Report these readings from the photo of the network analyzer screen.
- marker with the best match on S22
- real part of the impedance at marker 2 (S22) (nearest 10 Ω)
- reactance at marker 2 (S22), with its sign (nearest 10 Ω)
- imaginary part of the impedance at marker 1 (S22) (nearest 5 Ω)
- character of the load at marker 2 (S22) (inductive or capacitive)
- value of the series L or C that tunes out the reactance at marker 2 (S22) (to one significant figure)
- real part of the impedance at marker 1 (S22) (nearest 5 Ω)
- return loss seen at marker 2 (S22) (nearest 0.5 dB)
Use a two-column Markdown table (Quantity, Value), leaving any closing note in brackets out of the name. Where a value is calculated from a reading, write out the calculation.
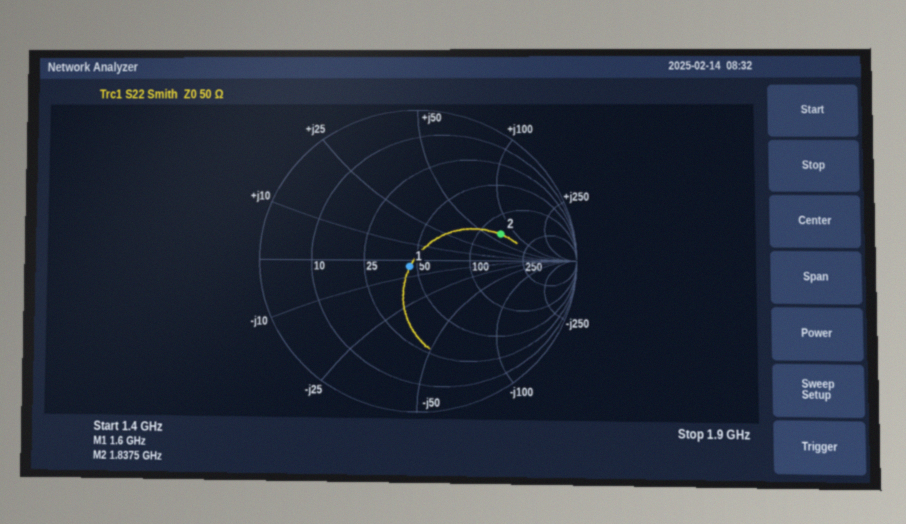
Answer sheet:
| Quantity | Value |
|---|---|
| marker with the best match on S22 | marker 1 |
| real part of the impedance at marker 2 (S22) | 140 Ω |
| reactance at marker 2 (S22), with its sign | +70 Ω |
| imaginary part of the impedance at marker 1 (S22) | -5 Ω |
| character of the load at marker 2 (S22) | inductive |
| value of the series L or C that tunes out the reactance at marker 2 (S22) | C = 1/(2π × 1.8375 GHz × 70 Ω) ≈ 1 pF |
| real part of the impedance at marker 1 (S22) | 45 Ω |
| return loss seen at marker 2 (S22) | 5.0 dB |
